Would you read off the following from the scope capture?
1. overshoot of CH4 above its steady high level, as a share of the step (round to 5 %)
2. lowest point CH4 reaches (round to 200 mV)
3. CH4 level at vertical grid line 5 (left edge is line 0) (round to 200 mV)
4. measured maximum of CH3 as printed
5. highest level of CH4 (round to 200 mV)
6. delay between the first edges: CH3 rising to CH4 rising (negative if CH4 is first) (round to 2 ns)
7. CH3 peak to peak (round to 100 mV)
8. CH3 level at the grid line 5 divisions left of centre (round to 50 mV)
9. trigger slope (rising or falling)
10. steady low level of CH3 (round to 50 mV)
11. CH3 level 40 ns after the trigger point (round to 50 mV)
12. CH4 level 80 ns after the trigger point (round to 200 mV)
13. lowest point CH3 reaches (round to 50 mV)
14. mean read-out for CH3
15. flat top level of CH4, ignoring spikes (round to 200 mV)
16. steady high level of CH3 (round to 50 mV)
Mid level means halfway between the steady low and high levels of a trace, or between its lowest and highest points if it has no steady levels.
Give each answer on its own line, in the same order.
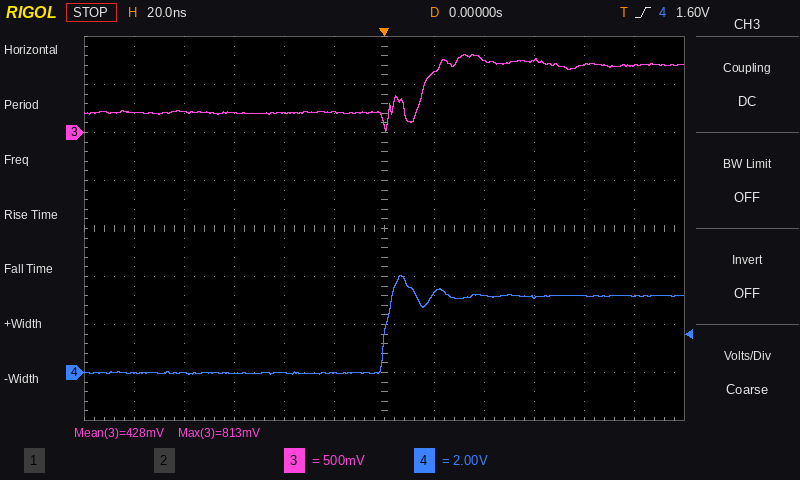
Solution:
25 %
0.0 V
0.0 V
813 mV
4.0 V
-16 ns
800 mV
200 mV
rising
200 mV
750 mV
3.2 V
0 mV
428 mV
3.2 V
700 mV
